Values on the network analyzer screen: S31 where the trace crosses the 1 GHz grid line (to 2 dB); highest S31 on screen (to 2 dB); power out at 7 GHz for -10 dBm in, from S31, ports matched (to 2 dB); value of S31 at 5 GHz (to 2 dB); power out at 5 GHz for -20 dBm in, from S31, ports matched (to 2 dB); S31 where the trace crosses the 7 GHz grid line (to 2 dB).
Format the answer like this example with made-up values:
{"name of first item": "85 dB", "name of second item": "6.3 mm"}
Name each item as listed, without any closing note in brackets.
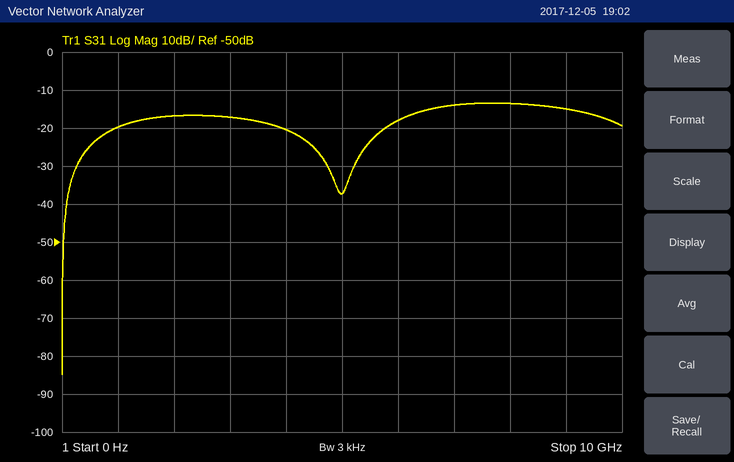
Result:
{"S31 where the trace crosses the 1 GHz grid line": "-20 dB", "highest S31 on screen": "-14 dB", "power out at 7 GHz for -10 dBm in, from S31, ports matched": "-24 dBm", "value of S31 at 5 GHz": "-38 dB", "power out at 5 GHz for -20 dBm in, from S31, ports matched": "-58 dBm", "S31 where the trace crosses the 7 GHz grid line": "-14 dB"}
